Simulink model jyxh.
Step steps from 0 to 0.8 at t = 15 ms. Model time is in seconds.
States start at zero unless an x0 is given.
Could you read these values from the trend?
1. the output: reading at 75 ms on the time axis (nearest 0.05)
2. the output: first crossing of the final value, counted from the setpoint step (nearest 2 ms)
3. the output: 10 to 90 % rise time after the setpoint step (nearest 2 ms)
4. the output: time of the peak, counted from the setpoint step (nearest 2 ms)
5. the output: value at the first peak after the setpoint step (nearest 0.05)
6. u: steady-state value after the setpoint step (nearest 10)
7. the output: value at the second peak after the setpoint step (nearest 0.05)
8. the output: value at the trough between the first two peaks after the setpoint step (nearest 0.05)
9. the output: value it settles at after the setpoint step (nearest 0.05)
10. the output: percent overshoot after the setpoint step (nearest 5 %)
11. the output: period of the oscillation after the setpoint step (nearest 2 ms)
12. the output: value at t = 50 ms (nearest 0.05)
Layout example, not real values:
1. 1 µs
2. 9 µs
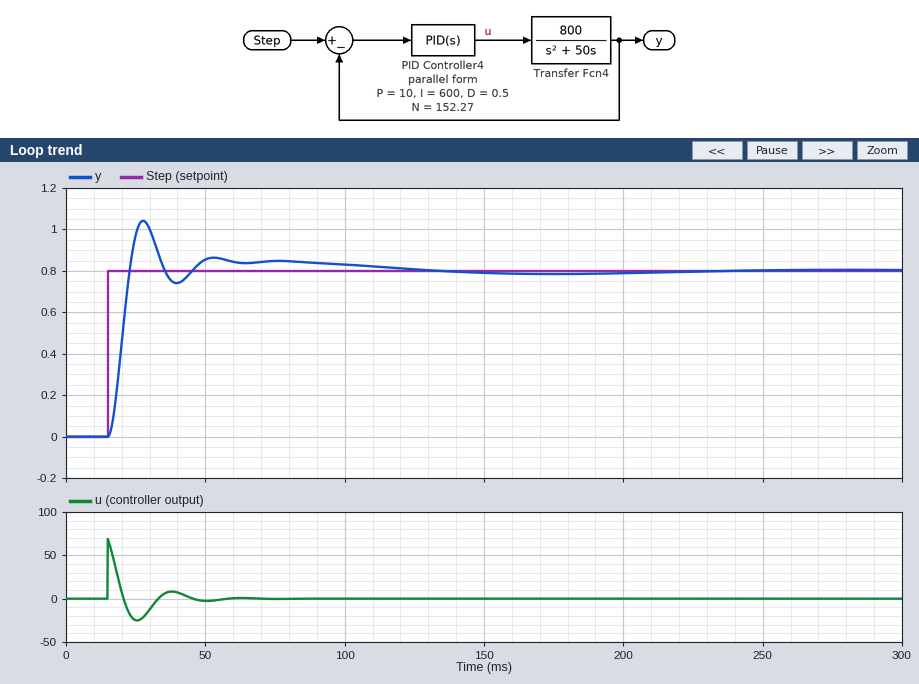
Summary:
1. 0.85
2. 8 ms
3. 6 ms
4. 12 ms
5. 1.05
6. 0
7. 0.85
8. 0.75
9. 0.80
10. 30 %
11. 26 ms
12. 0.85
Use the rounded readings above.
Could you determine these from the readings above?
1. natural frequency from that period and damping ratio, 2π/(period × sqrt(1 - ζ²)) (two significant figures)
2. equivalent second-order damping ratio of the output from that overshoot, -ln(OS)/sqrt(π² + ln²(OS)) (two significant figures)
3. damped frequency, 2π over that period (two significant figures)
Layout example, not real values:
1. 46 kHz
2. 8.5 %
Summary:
1. 0.26 rad/ms
2. 0.36
3. 0.24 rad/ms
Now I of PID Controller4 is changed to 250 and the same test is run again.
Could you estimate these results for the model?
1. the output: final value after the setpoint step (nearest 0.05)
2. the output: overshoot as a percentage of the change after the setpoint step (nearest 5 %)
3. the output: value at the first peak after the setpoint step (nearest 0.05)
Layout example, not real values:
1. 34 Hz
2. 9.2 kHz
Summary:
1. 0.80
2. 25 %
3. 1.00
